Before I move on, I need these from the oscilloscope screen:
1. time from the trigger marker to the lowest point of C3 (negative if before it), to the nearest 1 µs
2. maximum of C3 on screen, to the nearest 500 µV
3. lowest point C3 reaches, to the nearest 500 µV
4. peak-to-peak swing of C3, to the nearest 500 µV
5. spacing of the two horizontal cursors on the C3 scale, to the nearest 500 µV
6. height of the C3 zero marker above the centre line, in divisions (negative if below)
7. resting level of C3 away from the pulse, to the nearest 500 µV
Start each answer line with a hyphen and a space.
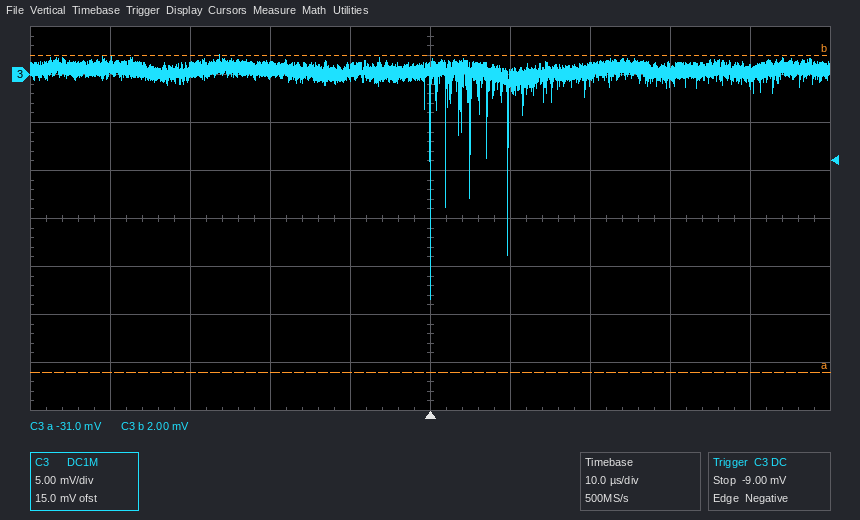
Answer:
- 0 µs
- 2.0 mV
- -23.5 mV
- 25.5 mV
- 33.0 mV
- +3.0 div
- 500 µV
